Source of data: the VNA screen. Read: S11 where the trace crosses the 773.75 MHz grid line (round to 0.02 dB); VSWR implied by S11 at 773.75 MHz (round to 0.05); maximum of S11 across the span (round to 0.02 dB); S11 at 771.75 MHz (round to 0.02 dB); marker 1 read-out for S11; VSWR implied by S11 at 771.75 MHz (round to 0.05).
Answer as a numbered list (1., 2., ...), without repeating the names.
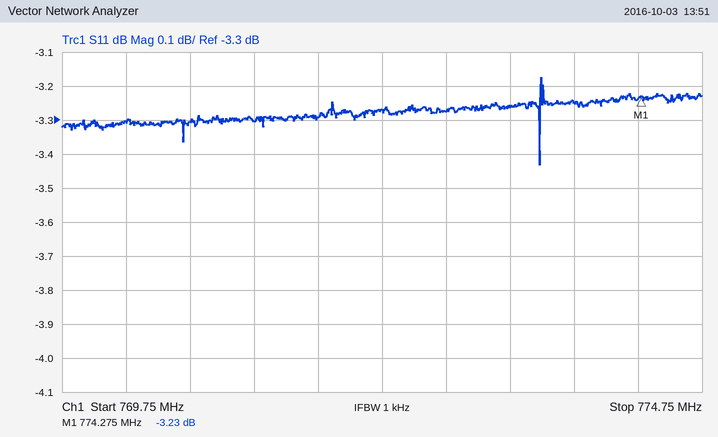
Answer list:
1. -3.24 dB
2. 5.40
3. -3.18 dB
4. -3.30 dB
5. -3.23 dB
6. 5.35
